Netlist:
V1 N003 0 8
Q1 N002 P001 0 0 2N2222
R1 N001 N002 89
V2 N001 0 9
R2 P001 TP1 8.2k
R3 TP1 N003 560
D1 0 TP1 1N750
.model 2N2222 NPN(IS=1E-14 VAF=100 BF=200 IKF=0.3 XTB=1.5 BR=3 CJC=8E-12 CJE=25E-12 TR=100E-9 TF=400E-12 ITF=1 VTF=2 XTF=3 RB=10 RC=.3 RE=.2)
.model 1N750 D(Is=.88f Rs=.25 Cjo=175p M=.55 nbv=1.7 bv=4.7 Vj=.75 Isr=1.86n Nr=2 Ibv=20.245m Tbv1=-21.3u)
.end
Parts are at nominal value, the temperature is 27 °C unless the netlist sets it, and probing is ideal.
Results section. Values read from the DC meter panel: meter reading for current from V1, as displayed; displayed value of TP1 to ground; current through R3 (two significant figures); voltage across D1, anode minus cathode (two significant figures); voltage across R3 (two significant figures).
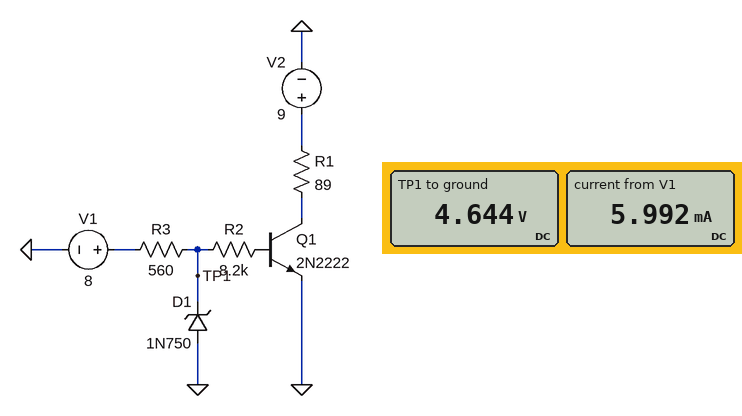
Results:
5.992 mA
4.644 V
6.0 mA
-4.6 V
3.4 V
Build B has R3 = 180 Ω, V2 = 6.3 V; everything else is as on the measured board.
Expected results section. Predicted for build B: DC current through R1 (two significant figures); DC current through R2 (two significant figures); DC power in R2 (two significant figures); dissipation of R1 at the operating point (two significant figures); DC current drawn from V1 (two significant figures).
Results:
69 mA
480 µA
1.9 mW
420 mW
18 mA
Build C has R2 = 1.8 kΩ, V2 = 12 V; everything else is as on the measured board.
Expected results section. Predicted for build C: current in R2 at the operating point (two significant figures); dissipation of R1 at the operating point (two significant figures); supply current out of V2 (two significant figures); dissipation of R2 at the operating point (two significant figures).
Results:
2.1 mA
1.6 W
130 mA
8.0 mW
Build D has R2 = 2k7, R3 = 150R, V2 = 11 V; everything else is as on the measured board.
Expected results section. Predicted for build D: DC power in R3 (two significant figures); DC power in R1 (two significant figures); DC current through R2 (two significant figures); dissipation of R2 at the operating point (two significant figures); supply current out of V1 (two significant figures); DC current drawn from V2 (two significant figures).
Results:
72 mW
1.3 W
1.4 mA
5.6 mW
22 mA
120 mA
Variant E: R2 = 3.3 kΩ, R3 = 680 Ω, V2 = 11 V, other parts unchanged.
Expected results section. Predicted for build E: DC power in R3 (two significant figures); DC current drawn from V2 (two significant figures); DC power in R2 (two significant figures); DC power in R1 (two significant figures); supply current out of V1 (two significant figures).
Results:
17 mW
120 mA
4.4 mW
1.3 W
5.0 mA
